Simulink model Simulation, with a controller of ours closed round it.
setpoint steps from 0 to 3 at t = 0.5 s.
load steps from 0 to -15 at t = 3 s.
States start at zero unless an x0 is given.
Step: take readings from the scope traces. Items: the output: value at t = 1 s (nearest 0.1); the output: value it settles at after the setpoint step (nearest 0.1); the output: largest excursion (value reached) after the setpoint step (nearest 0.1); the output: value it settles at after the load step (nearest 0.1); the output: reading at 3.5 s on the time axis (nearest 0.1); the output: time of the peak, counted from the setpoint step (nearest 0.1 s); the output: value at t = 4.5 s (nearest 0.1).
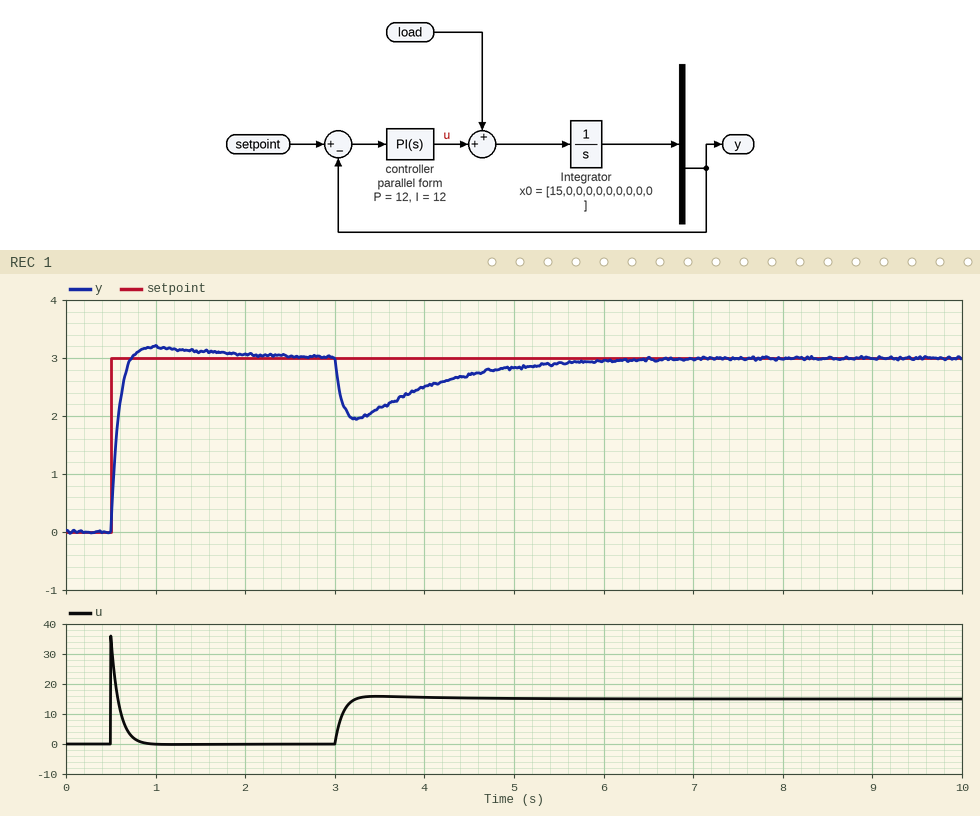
3.2
3.0
3.2
3.0
2.1
0.5 s
2.7
